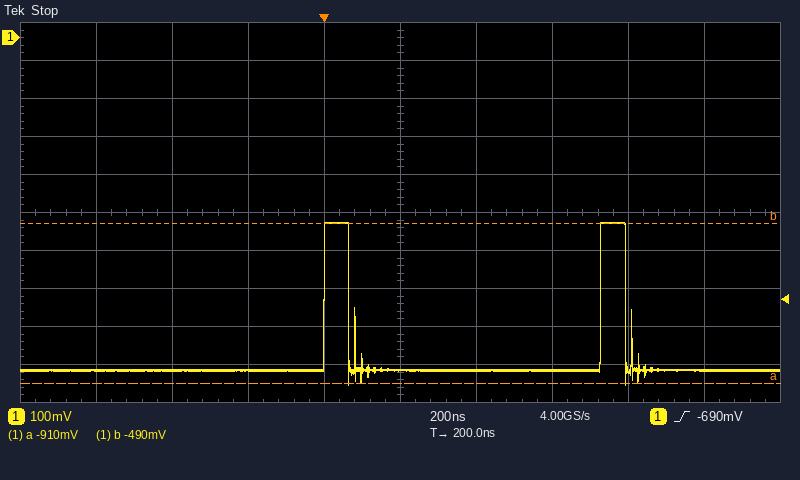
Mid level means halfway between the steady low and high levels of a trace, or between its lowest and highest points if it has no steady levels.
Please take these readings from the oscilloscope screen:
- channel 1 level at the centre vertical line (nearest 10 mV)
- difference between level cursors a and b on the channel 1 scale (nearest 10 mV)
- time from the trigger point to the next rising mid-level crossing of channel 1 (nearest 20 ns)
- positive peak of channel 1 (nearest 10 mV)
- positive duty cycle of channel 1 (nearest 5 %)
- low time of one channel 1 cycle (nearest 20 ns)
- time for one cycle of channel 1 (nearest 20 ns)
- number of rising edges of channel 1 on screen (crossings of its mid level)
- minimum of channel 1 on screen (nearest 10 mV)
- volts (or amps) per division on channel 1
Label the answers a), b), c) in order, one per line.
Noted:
a) -870 mV
b) 420 mV
c) 720 ns
d) -490 mV
e) 10 %
f) 660 ns
g) 720 ns
h) 2
i) -910 mV
j) 100 mV
